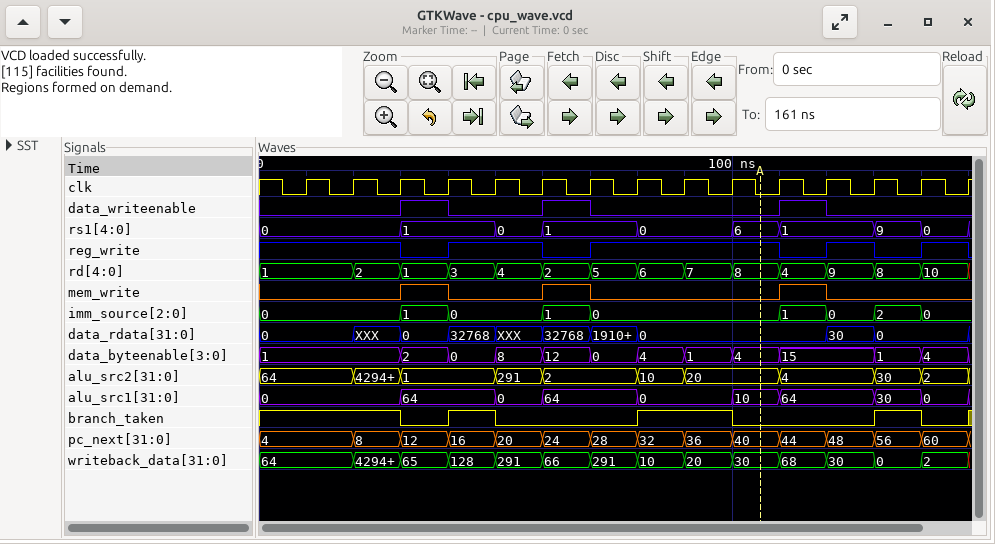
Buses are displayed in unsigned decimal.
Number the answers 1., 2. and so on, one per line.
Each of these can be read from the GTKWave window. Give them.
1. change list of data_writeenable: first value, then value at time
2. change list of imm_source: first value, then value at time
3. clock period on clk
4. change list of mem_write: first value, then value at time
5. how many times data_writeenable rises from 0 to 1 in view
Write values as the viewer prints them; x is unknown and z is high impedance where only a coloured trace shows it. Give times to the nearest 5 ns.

1. 0, 1 at 30 ns, 0 at 40 ns, 1 at 60 ns, 0 at 70 ns, 1 at 110 ns, 0 at 120 ns
2. 0, 1 at 30 ns, 0 at 40 ns, 1 at 60 ns, 0 at 70 ns, 1 at 110 ns, 0 at 120 ns, 2 at 130 ns, 0 at 140 ns
3. 10 ns
4. 0, 1 at 30 ns, 0 at 40 ns, 1 at 60 ns, 0 at 70 ns, 1 at 110 ns, 0 at 120 ns
5. 3
